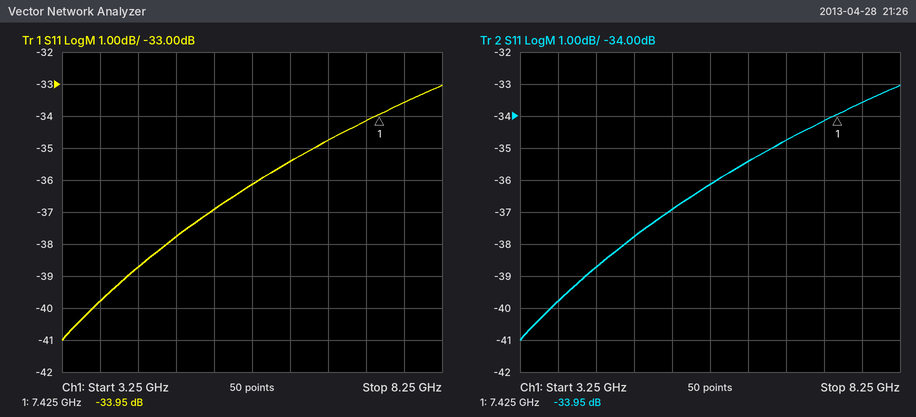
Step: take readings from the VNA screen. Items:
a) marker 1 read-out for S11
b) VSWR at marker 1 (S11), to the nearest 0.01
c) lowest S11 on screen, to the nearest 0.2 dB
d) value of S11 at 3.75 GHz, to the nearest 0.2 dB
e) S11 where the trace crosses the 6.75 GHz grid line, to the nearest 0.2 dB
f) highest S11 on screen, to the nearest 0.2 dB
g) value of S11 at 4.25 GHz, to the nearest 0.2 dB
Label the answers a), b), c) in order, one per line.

a) -33.95 dB
b) 1.04
c) -41.0 dB
d) -39.8 dB
e) -34.8 dB
f) -33.0 dB
g) -38.8 dB
